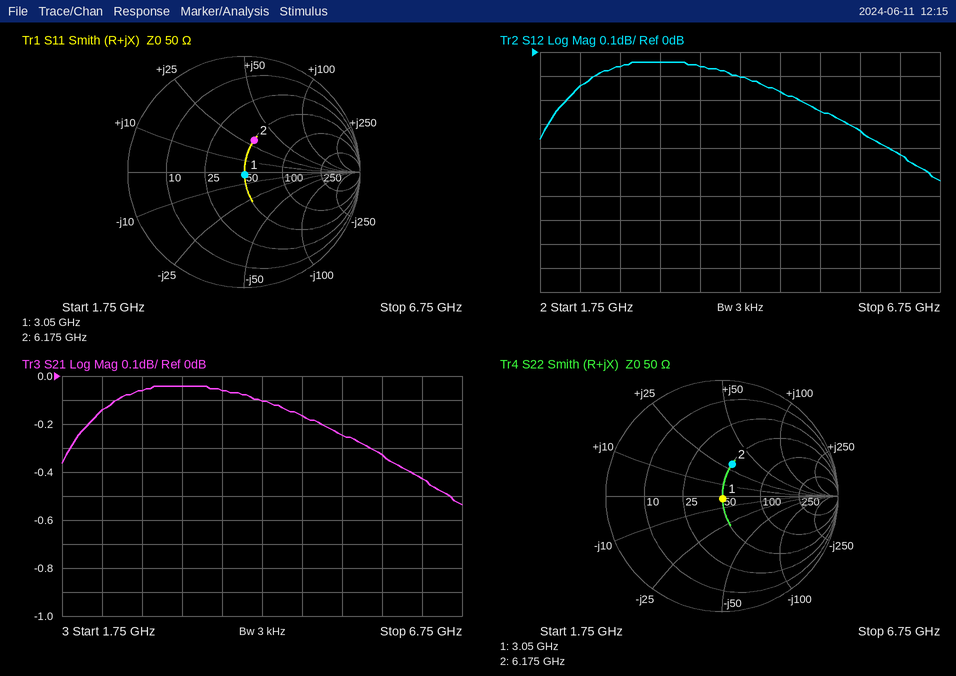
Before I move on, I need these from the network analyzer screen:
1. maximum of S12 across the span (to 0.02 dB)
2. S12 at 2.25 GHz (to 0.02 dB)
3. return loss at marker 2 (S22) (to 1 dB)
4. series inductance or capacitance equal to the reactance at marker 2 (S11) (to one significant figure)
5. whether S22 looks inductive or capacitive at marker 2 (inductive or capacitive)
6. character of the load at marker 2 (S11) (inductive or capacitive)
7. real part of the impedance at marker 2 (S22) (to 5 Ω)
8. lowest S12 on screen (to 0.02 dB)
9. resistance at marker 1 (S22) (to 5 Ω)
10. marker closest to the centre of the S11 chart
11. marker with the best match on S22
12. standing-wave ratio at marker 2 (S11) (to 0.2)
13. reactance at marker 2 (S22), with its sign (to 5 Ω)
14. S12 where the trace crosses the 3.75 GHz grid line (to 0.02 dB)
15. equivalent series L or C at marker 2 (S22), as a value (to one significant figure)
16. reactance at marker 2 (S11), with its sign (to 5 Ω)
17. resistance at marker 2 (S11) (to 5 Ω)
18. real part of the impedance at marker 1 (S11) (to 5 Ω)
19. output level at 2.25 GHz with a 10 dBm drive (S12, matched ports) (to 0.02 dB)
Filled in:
-0.04 dB
-0.14 dB
11 dB
800 pH
inductive
inductive
50 Ω
-0.54 dB
50 Ω
marker 1
marker 1
1.8
+30 Ω
-0.06 dB
800 pH
+30 Ω
50 Ω
50 Ω
9.86 dBm
